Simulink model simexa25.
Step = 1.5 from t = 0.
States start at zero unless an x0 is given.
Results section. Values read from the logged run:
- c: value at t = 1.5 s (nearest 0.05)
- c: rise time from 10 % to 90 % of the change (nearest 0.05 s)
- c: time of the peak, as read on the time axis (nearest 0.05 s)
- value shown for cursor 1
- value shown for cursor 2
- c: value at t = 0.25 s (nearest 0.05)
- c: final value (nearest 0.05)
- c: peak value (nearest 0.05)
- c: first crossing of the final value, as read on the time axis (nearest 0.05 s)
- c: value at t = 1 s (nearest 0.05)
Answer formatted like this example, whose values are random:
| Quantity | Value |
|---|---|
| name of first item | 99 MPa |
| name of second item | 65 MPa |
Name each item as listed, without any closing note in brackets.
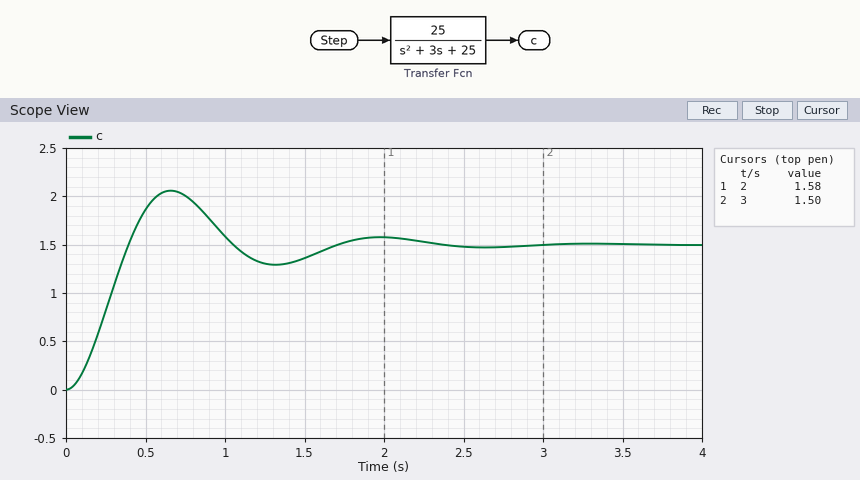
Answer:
| Quantity | Value |
|---|---|
| c: value at t = 1.5 s | 1.35 |
| c: rise time from 10 % to 90 % of the change | 0.25 s |
| c: time of the peak, as read on the time axis | 0.65 s |
| value shown for cursor 1 | 1.58 |
| value shown for cursor 2 | 1.50 |
| c: value at t = 0.25 s | 0.80 |
| c: final value | 1.50 |
| c: peak value | 2.05 |
| c: first crossing of the final value, as read on the time axis | 0.40 s |
| c: value at t = 1 s | 1.60 |
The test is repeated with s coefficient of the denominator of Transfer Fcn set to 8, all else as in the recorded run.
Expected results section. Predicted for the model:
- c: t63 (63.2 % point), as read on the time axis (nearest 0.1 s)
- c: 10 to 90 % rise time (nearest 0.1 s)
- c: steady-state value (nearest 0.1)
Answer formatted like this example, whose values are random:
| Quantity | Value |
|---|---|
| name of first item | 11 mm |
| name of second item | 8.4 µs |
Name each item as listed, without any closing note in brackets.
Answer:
| Quantity | Value |
|---|---|
| c: t63 (63.2 % point), as read on the time axis | 0.4 s |
| c: 10 to 90 % rise time | 0.5 s |
| c: steady-state value | 1.5 |
